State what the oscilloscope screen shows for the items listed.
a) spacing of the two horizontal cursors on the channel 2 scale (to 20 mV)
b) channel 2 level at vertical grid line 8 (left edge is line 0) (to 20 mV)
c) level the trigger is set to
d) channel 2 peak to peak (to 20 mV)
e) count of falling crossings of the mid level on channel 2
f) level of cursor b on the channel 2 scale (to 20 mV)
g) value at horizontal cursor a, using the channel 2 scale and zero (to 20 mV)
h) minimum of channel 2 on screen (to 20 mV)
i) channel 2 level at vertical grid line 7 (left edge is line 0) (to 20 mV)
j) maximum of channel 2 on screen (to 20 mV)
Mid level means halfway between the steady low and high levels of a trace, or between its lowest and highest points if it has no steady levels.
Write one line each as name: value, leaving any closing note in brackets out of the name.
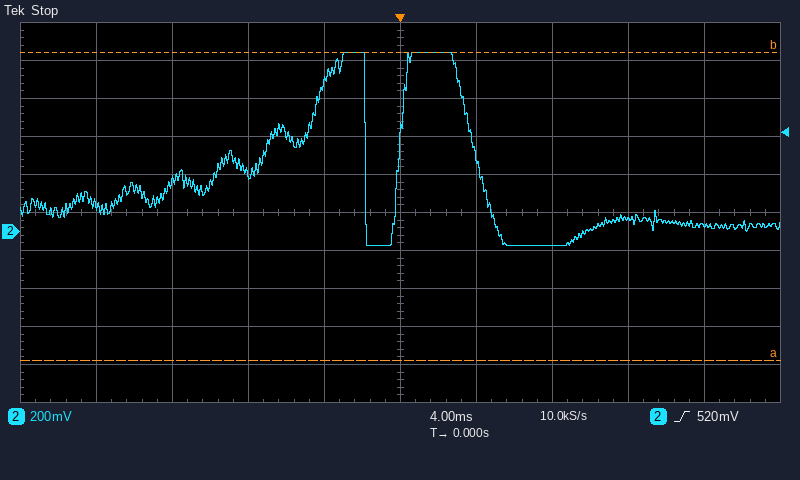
spacing of the two horizontal cursors on the channel 2 scale: 1.62 V
channel 2 level at vertical grid line 8 (left edge is line 0): 60 mV
level the trigger is set to: 520 mV
channel 2 peak to peak: 1.02 V
count of falling crossings of the mid level on channel 2: 2
level of cursor b on the channel 2 scale: 940 mV
value at horizontal cursor a, using the channel 2 scale and zero: -680 mV
minimum of channel 2 on screen: -80 mV
channel 2 level at vertical grid line 7 (left edge is line 0): -80 mV
maximum of channel 2 on screen: 940 mV
